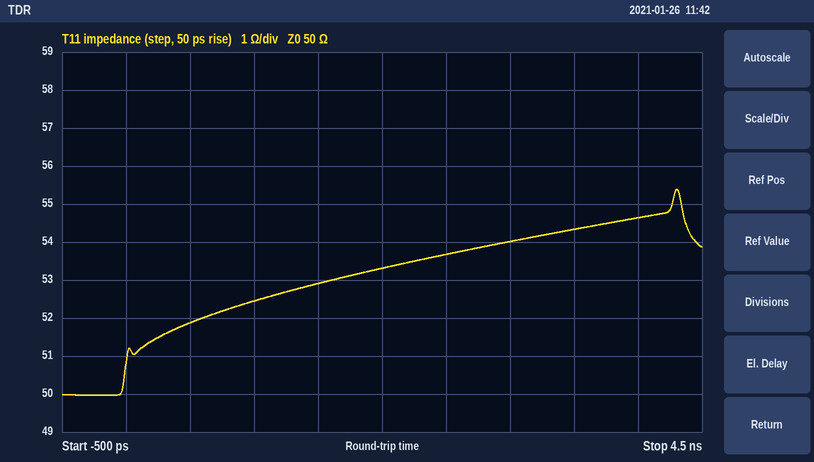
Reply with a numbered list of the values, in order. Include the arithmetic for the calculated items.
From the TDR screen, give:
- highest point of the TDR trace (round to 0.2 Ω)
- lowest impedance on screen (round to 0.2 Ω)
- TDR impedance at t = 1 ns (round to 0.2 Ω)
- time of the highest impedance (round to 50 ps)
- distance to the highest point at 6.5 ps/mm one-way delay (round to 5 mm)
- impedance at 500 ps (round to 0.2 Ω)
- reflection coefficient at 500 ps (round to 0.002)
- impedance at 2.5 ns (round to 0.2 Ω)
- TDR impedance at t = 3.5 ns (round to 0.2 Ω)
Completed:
1. 55.4 Ω
2. 50.0 Ω
3. 52.4 Ω
4. 4.30 ns
5. 4.30 ns / 2 / 6.5 ps/mm ≈ 331 mm, so 330 mm to the nearest 5 mm
6. 51.8 Ω
7. (51.8 − 50)/(51.8 + 50) ≈ +0.018
8. 53.6 Ω
9. 54.4 Ω
